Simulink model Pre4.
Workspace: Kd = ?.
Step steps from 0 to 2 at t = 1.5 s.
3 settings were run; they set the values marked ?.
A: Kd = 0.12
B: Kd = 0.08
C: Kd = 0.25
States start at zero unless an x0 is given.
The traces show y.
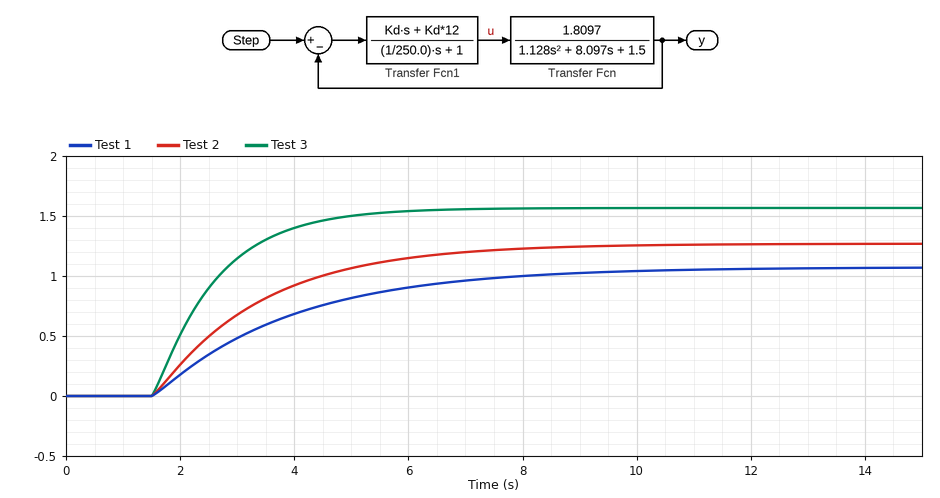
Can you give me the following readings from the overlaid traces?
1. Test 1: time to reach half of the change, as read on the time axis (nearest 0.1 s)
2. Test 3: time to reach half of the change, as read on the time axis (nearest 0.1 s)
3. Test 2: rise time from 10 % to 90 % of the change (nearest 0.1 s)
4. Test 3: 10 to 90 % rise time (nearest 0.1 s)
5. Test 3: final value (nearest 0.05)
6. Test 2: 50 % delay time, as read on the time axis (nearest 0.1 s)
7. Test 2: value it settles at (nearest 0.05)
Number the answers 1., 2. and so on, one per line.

1. 3.2 s
2. 2.3 s
3. 4.1 s
4. 2.4 s
5. 1.55
6. 2.9 s
7. 1.25
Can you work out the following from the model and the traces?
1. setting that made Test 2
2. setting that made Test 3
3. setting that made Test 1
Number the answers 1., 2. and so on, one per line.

1. A
2. C
3. B
